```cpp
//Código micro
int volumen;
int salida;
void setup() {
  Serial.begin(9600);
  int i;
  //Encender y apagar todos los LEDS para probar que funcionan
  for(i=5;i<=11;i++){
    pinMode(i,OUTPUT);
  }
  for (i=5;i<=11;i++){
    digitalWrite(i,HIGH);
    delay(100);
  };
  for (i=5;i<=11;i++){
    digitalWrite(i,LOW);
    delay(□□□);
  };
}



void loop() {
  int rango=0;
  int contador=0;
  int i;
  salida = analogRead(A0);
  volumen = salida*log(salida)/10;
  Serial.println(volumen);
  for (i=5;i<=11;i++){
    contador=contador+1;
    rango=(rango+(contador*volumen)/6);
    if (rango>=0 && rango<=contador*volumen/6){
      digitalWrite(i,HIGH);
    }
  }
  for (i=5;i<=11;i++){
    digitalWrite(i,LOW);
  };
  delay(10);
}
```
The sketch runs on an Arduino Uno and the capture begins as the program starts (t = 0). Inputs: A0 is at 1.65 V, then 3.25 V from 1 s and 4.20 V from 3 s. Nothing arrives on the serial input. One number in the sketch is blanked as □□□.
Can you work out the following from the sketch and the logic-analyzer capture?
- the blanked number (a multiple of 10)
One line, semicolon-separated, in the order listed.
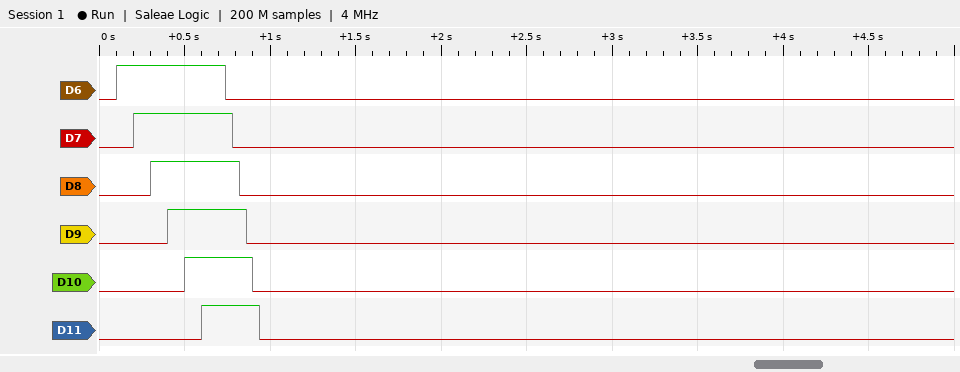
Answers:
40
